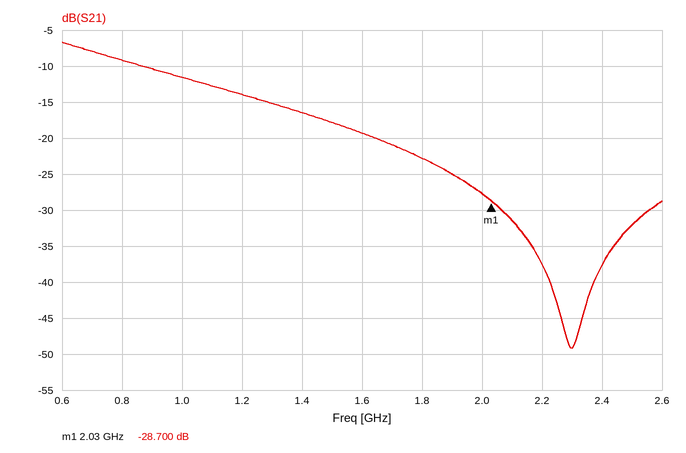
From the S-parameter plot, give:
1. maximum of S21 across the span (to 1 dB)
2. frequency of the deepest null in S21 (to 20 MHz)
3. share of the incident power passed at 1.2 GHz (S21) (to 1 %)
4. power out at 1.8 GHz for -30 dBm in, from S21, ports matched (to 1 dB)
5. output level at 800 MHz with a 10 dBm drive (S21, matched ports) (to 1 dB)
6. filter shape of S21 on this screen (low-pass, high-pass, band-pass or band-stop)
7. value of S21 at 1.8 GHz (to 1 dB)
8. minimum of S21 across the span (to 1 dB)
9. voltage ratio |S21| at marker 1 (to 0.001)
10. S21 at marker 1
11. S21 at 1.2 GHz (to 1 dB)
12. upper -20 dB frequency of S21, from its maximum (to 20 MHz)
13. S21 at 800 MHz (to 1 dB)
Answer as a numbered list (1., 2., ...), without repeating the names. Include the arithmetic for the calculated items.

1. -7 dB
2. 2.30 GHz
3. 10^(-14/10) ≈ 4 %
4. -30 dBm + (-23 dB) = -53 dBm
5. 10 dBm + (-9 dB) = 1 dBm
6. low-pass
7. -23 dB
8. -49 dB
9. 10^(-28.7/20) ≈ 0.037
10. -28.700 dB
11. -14 dB
12. 1.96 GHz
13. -9 dB
